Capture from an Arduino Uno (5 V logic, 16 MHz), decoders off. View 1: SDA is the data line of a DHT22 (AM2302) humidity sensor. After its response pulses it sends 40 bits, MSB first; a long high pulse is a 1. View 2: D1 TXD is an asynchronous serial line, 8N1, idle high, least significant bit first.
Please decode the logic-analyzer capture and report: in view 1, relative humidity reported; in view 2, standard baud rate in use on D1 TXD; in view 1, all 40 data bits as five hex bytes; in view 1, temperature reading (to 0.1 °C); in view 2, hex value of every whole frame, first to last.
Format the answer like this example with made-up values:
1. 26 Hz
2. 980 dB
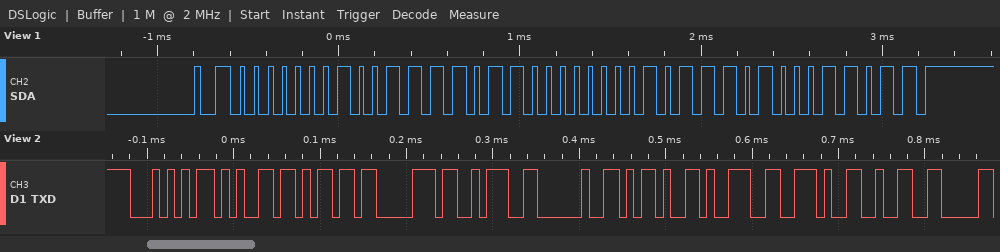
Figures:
1. 31.7 %
2. 115200 baud
3. 01 3D 80 5D 1B
4. -9.3 °C
5. 54 65 6D 70 3A 20 2D 39 2E 32
